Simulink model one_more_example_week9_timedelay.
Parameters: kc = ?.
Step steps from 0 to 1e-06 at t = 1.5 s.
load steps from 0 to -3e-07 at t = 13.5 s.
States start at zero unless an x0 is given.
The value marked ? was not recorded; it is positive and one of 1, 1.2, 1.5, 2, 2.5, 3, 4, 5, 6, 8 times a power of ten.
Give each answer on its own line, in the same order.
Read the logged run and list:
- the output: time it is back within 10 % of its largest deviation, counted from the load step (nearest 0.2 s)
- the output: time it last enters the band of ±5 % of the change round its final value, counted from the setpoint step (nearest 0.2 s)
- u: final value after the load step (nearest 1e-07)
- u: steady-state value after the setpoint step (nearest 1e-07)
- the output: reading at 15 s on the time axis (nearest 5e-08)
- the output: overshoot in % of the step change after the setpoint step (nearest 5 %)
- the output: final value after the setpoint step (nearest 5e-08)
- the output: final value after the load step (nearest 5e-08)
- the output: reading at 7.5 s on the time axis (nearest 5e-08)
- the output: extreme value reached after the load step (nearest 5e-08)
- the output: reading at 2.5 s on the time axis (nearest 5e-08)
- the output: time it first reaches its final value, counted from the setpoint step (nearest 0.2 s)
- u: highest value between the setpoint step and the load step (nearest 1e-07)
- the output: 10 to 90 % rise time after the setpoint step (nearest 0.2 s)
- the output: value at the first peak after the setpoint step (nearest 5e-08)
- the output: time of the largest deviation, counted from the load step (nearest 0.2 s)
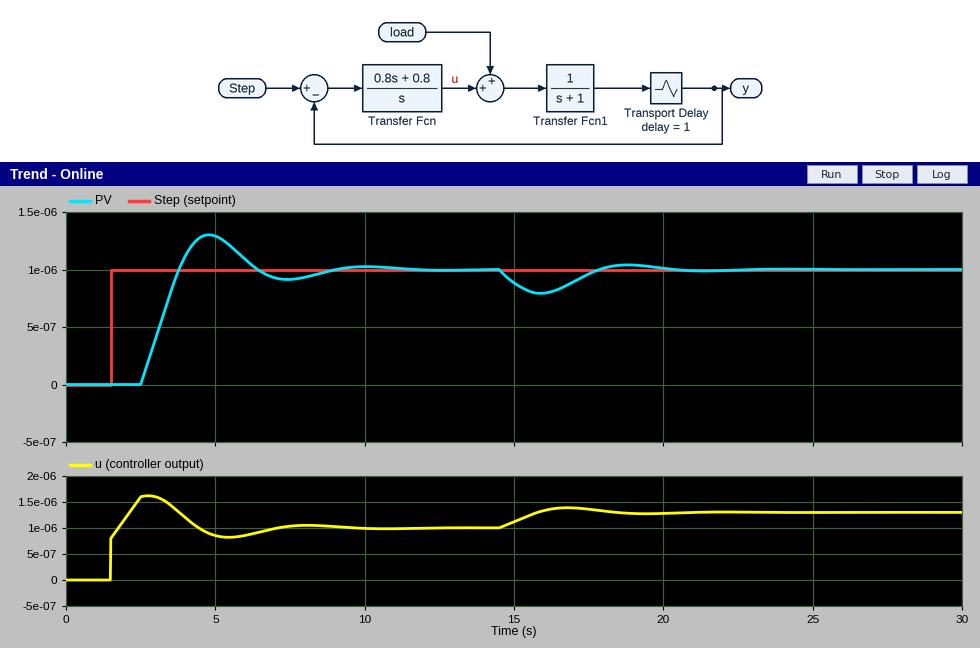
6.2 s
6.8 s
0.0000013
0.0000010
0.00000090
30 %
0.00000100
0.00000100
0.00000090
0.00000080
0.00000000
2.2 s
0.0000016
1.0 s
0.00000130
2.4 s
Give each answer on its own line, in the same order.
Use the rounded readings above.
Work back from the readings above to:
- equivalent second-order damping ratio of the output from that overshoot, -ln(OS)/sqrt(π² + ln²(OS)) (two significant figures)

0.36
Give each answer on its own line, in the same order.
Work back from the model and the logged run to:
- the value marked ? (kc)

0.8
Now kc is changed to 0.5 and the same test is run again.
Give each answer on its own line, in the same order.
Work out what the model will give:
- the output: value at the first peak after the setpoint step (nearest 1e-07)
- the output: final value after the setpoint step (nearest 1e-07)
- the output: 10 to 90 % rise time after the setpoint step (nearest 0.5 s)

0.0000010
0.0000010
2.0 s
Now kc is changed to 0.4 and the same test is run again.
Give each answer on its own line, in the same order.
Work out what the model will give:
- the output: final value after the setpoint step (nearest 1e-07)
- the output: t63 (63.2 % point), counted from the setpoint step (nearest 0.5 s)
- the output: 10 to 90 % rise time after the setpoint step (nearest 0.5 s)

0.0000010
2.5 s
3.0 s
